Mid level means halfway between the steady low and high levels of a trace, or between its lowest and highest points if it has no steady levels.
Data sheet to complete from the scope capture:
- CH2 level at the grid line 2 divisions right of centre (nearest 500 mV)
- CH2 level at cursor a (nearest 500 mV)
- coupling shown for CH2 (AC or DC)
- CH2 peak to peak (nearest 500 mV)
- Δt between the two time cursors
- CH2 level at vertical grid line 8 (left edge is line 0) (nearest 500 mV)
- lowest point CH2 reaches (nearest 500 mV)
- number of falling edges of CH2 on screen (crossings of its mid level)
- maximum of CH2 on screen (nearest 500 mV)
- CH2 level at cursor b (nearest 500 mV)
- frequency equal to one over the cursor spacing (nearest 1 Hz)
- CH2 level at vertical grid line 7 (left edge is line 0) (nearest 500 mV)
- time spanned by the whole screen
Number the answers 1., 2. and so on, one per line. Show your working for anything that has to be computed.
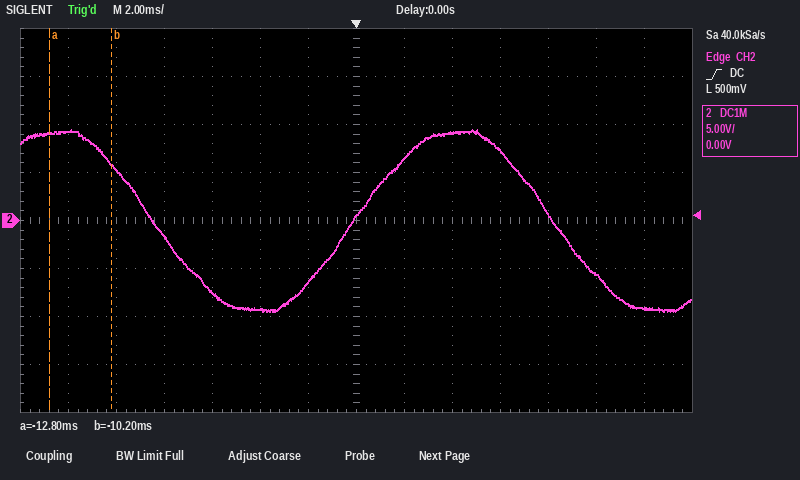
1. 9.0 V
2. 9.0 V
3. DC
4. 9.5 V − (-9.5 V) = 19.0 V
5. -10.2 ms − (-12.8 ms) = 2.6 ms
6. 6.5 V
7. -9.5 V
8. 2
9. 9.5 V
10. 6.0 V
11. 1 / 2.6 ms ≈ 385 Hz
12. 500 mV
13. 28 ms
